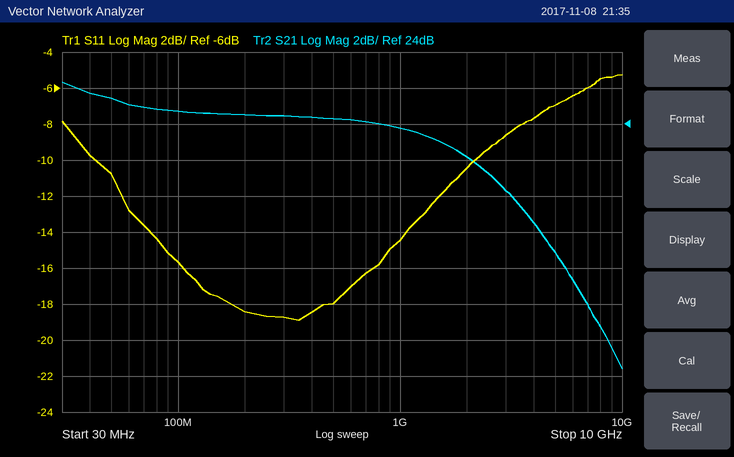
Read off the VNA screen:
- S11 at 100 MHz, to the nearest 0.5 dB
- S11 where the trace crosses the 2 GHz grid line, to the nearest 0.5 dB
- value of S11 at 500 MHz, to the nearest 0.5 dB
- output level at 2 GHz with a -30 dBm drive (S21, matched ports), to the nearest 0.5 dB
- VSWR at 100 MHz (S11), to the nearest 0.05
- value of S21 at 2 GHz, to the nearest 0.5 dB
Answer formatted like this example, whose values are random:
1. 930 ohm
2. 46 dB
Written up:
1. -15.5 dB
2. -10.5 dB
3. -18.0 dB
4. -8.0 dBm
5. 1.40
6. 22.0 dB
